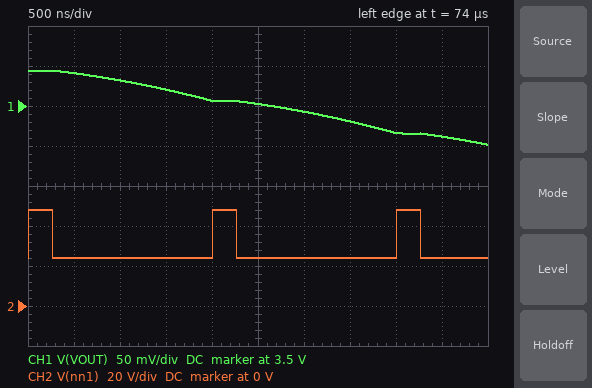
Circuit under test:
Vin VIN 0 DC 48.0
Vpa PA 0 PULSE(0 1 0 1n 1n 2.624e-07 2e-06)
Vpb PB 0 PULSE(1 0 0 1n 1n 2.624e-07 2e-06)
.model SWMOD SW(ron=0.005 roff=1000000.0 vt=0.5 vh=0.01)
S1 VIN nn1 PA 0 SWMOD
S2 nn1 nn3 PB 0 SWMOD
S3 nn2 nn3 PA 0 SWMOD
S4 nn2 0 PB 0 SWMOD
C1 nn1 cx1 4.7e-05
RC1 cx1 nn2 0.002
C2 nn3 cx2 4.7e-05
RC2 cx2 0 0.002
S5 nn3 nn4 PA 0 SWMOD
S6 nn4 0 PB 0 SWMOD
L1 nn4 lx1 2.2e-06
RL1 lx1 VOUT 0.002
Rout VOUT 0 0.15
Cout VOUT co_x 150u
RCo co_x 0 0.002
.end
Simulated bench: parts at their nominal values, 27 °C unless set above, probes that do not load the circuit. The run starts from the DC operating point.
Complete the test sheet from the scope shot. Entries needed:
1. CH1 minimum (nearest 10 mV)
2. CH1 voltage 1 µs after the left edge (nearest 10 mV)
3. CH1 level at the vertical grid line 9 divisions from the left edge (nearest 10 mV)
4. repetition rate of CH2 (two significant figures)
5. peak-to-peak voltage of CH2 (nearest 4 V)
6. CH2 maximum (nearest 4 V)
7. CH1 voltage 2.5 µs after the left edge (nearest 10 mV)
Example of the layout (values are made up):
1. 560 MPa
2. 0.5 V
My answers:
1. 3.45 V
2. 3.53 V
3. 3.46 V
4. 500 kHz
5. 24 V
6. 48 V
7. 3.50 V
